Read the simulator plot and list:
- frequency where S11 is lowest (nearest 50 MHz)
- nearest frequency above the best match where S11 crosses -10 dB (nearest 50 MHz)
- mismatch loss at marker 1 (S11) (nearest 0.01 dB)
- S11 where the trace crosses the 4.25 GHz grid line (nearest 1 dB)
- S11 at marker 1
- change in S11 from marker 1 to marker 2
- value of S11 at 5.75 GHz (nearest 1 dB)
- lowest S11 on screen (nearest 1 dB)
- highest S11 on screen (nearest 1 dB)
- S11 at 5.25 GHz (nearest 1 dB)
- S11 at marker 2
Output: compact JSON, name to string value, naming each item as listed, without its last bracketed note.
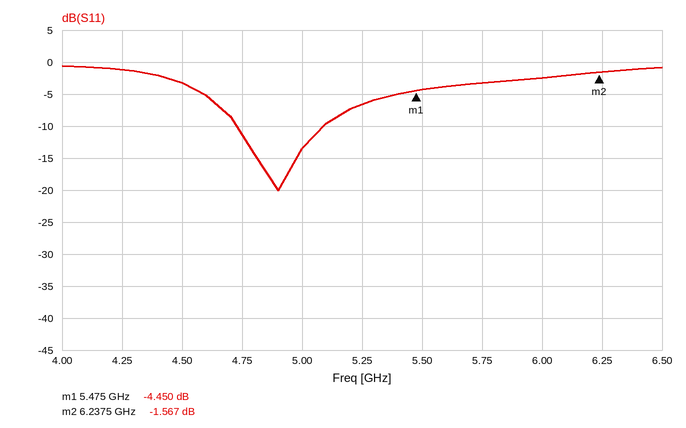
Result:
{"frequency where S11 is lowest": "4.90 GHz", "nearest frequency above the best match where S11 crosses -10 dB": "5.10 GHz", "mismatch loss at marker 1 (S11)": "1.93 dB", "S11 where the trace crosses the 4.25 GHz grid line": "-1 dB", "S11 at marker 1": "-4.450 dB", "change in S11 from marker 1 to marker 2": "2.883 dB", "value of S11 at 5.75 GHz": "-3 dB", "lowest S11 on screen": "-20 dB", "highest S11 on screen": "-1 dB", "S11 at 5.25 GHz": "-7 dB", "S11 at marker 2": "-1.567 dB"}
